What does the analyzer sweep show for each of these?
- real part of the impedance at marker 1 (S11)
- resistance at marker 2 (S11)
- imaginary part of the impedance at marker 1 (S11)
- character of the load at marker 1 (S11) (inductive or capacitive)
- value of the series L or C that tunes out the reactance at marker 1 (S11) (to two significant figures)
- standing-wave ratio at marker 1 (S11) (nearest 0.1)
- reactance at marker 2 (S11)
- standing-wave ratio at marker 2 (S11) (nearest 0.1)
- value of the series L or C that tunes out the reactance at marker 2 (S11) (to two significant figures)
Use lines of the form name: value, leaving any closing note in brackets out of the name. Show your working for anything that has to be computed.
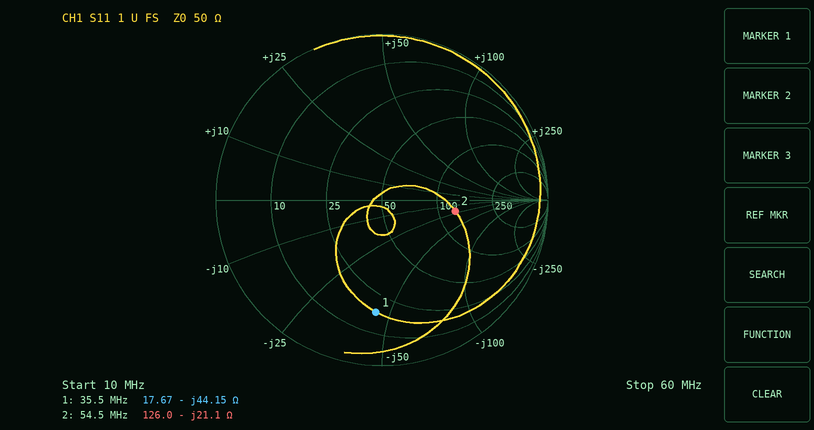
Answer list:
real part of the impedance at marker 1: 17.67 Ω
resistance at marker 2: 126.0 Ω
imaginary part of the impedance at marker 1: -44.15 Ω
character of the load at marker 1 (S11): capacitive
value of the series L or C that tunes out the reactance at marker 1 (S11): L = 44.15 Ω/(2π × 35.5 MHz) ≈ 198 nH, so 200 nH to two significant figures
standing-wave ratio at marker 1 (S11): 5.2
reactance at marker 2: -21.1 Ω
standing-wave ratio at marker 2 (S11): 2.6
value of the series L or C that tunes out the reactance at marker 2 (S11): L = 21.1 Ω/(2π × 54.5 MHz) ≈ 62 nH
